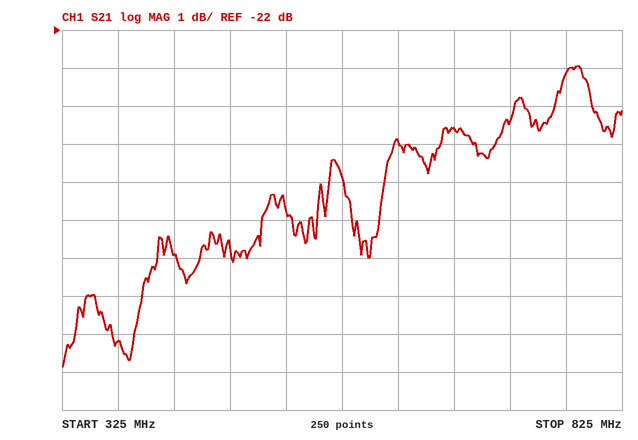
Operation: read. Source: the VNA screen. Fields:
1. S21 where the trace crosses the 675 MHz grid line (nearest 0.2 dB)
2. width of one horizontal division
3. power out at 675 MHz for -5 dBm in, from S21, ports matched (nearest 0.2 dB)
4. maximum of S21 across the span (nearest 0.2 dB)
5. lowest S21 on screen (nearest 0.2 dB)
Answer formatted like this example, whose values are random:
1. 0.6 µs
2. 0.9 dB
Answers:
1. -24.6 dB
2. 50 MHz
3. -29.6 dBm
4. -23.0 dB
5. -30.8 dB
